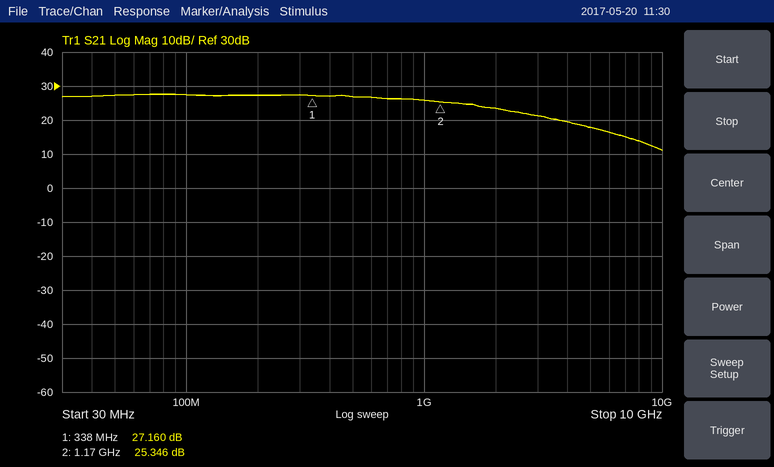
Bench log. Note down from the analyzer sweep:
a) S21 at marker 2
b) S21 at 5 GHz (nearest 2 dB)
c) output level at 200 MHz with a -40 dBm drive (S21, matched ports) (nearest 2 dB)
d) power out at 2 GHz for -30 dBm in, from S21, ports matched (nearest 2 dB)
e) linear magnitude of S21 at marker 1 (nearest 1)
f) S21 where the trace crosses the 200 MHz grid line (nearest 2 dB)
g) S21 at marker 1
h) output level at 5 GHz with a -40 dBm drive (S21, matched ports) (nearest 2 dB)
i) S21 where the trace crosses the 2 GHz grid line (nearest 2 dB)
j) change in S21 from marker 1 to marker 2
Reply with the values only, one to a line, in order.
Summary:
25.346 dB
18 dB
-12 dBm
-6 dBm
23
28 dB
27.160 dB
-22 dBm
24 dB
-1.814 dB
